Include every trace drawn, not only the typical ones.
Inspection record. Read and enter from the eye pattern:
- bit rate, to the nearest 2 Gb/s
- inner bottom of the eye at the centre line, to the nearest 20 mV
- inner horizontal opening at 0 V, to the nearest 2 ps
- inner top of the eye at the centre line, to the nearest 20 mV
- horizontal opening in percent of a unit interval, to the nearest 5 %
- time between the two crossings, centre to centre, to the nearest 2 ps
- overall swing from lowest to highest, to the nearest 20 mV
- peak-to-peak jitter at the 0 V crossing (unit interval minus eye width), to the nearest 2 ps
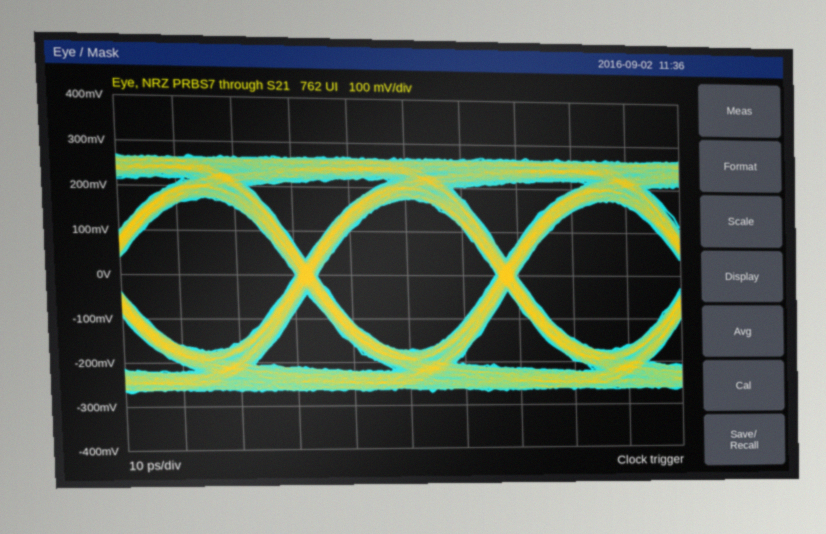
28 Gb/s
-180 mV
32 ps
180 mV
90 %
36 ps
540 mV
4 ps
